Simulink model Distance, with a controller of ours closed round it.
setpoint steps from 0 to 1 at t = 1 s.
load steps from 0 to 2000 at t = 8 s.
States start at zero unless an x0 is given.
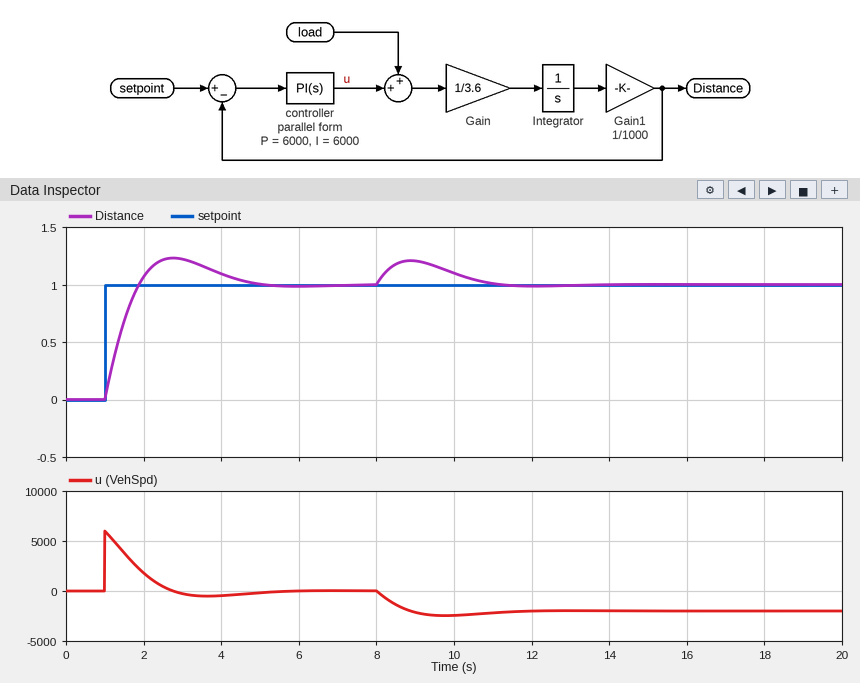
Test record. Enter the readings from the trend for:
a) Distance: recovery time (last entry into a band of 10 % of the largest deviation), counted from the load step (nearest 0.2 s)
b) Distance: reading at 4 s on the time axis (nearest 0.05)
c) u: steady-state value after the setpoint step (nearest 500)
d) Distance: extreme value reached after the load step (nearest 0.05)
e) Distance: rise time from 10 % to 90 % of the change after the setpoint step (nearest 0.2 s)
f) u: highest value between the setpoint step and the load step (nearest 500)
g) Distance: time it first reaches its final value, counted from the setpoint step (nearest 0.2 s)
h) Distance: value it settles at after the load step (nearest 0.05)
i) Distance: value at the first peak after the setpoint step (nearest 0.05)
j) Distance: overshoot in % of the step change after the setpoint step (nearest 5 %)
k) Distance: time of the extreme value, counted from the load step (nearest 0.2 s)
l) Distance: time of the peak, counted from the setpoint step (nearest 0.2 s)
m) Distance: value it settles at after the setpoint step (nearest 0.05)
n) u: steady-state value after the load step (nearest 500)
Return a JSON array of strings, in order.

["2.8 s", "1.10", "0", "1.20", "0.6 s", "6000", "0.8 s", "1.00", "1.25", "25 %", "0.8 s", "1.8 s", "1.00", "-2000"]
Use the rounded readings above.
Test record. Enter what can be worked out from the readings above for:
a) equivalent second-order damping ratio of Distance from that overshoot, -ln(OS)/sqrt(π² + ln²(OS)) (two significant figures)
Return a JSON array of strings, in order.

["0.40"]
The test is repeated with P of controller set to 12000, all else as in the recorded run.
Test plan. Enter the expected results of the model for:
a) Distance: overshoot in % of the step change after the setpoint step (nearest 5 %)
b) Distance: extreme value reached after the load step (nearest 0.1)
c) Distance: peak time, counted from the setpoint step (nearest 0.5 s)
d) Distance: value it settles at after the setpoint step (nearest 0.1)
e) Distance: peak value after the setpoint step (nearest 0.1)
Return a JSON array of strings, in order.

["10 %", "1.1", "1.5 s", "1.0", "1.1"]
